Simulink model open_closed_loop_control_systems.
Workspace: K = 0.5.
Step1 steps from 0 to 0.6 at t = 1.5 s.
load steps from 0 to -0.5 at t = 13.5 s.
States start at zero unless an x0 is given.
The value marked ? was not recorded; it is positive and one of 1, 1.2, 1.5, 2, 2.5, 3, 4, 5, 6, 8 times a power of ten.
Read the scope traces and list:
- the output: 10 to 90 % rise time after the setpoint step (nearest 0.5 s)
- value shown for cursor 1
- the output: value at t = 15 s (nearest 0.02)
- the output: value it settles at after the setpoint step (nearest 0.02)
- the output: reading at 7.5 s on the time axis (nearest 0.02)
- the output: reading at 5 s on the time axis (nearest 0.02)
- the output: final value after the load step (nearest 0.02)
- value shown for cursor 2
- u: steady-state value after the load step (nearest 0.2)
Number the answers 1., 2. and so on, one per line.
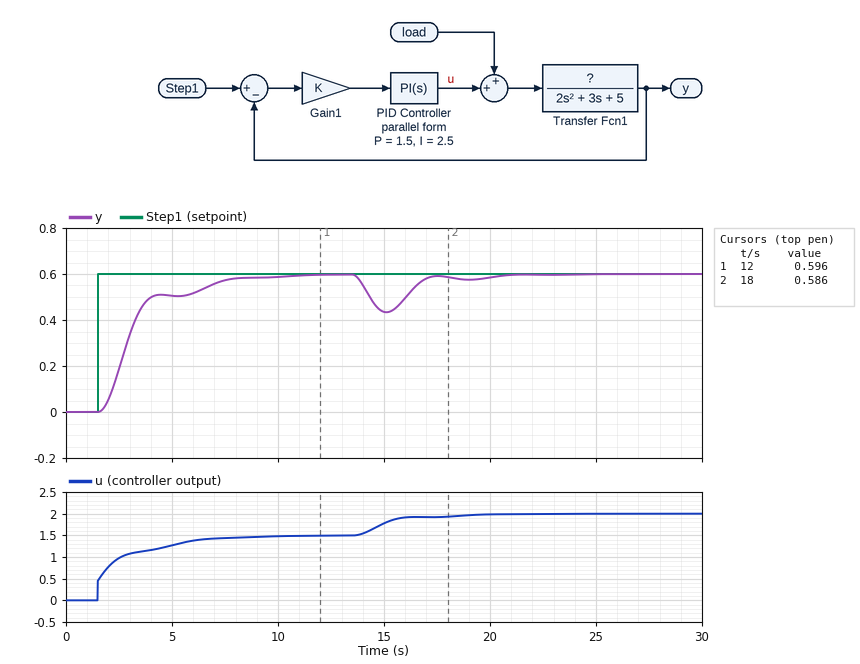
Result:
1. 4.5 s
2. 0.596
3. 0.44
4. 0.60
5. 0.58
6. 0.50
7. 0.60
8. 0.586
9. 2.0
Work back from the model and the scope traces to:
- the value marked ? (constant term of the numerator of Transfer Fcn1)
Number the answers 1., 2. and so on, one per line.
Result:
1. 2
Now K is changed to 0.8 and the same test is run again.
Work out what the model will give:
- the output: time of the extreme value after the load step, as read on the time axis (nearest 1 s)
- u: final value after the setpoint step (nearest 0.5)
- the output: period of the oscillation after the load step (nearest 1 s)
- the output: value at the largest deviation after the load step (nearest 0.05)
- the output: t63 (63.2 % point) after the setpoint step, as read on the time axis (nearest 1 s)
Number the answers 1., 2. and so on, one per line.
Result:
1. 15 s
2. 1.5
3. 4 s
4. 0.45
5. 3 s
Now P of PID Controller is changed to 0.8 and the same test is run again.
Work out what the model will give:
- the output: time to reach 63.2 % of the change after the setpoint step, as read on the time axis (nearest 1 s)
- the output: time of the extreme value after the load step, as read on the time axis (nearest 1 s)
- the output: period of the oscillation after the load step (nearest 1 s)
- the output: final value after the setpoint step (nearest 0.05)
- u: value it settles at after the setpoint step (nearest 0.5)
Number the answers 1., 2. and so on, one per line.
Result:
1. 3 s
2. 15 s
3. 4 s
4. 0.60
5. 1.5
